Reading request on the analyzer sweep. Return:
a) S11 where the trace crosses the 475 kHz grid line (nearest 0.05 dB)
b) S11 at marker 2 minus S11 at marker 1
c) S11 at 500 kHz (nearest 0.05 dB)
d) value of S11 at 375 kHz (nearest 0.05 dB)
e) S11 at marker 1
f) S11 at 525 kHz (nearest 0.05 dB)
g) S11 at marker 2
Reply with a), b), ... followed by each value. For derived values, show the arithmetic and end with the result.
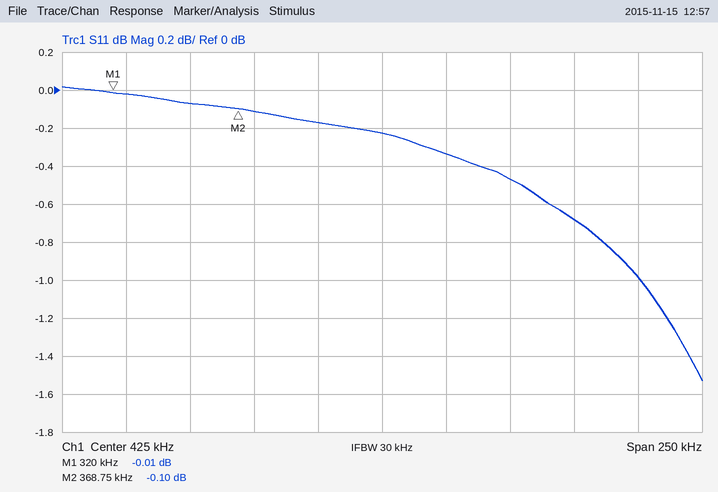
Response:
a) -0.45 dB
b) -0.1 − (-0.01) = -0.09 dB
c) -0.70 dB
d) -0.10 dB
e) -0.01 dB
f) -1.00 dB
g) -0.10 dB
